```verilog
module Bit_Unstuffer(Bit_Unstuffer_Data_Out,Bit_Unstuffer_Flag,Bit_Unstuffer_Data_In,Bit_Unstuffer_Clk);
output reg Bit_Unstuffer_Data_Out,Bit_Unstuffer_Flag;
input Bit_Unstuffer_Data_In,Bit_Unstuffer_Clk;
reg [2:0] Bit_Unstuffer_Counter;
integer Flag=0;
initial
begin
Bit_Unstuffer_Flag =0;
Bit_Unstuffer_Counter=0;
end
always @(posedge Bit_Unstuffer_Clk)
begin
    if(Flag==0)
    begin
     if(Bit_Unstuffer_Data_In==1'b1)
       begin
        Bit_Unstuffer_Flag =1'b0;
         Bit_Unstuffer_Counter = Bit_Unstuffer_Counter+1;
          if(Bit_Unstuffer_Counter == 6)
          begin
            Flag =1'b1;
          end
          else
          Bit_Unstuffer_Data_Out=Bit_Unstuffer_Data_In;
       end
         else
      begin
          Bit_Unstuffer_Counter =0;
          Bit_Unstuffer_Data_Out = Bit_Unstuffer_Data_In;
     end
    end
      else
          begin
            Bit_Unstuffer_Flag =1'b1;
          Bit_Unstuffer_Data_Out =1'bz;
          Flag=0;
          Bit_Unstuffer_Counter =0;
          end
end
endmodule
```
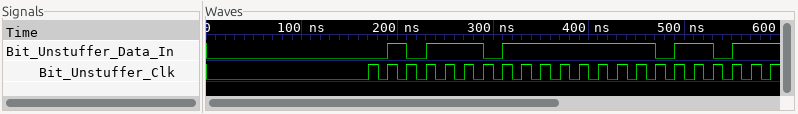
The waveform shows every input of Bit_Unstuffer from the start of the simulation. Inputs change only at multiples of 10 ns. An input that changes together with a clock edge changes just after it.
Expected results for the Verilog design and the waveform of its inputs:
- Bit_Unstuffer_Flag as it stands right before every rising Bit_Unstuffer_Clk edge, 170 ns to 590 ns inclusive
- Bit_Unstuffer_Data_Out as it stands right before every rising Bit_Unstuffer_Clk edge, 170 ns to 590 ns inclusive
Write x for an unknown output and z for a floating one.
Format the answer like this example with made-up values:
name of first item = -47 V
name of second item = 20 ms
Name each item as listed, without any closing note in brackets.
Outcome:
Bit_Unstuffer_Flag as it stands right before every rising Bit_Unstuffer_Clk edge, 170 ns to 590 ns inclusive = 0 0 0 0 0 0 0 0 0 0 0 0 0 0 0 1 0 0 0 0 0 0
Bit_Unstuffer_Data_Out as it stands right before every rising Bit_Unstuffer_Clk edge, 170 ns to 590 ns inclusive = x 0 0 1 0 1 1 1 0 1 1 1 1 1 1 z 1 0 1 1 0 1
